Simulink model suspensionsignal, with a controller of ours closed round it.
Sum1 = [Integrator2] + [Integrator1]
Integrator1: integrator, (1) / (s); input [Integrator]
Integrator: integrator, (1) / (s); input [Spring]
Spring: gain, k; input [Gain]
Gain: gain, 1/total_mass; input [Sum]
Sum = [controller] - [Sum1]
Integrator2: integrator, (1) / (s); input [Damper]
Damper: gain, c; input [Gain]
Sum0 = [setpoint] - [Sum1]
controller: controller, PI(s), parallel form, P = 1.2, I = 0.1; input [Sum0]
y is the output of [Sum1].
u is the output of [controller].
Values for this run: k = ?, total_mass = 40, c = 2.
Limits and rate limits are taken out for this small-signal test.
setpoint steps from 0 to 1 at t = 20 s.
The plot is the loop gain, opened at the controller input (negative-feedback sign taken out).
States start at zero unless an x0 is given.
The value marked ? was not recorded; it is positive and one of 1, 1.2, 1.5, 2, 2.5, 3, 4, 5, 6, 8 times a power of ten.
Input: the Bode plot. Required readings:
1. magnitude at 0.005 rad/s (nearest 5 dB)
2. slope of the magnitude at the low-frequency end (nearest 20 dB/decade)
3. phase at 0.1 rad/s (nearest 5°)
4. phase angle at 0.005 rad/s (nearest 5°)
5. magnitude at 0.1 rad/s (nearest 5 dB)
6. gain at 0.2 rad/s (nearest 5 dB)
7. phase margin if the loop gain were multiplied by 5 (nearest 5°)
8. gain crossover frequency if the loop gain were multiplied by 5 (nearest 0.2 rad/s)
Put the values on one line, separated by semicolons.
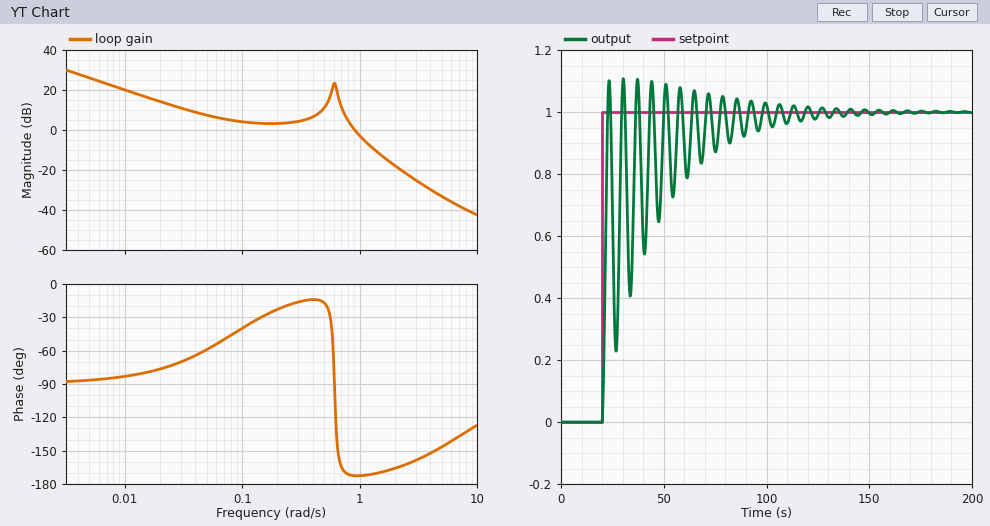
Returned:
25 dB; -20 dB/decade; -40°; -85°; 5 dB; 5 dB; 10°; 1.6 rad/s
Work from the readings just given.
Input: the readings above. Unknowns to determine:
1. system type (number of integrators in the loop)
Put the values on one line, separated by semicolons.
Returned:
1
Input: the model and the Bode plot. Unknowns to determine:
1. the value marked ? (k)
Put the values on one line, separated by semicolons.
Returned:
15
